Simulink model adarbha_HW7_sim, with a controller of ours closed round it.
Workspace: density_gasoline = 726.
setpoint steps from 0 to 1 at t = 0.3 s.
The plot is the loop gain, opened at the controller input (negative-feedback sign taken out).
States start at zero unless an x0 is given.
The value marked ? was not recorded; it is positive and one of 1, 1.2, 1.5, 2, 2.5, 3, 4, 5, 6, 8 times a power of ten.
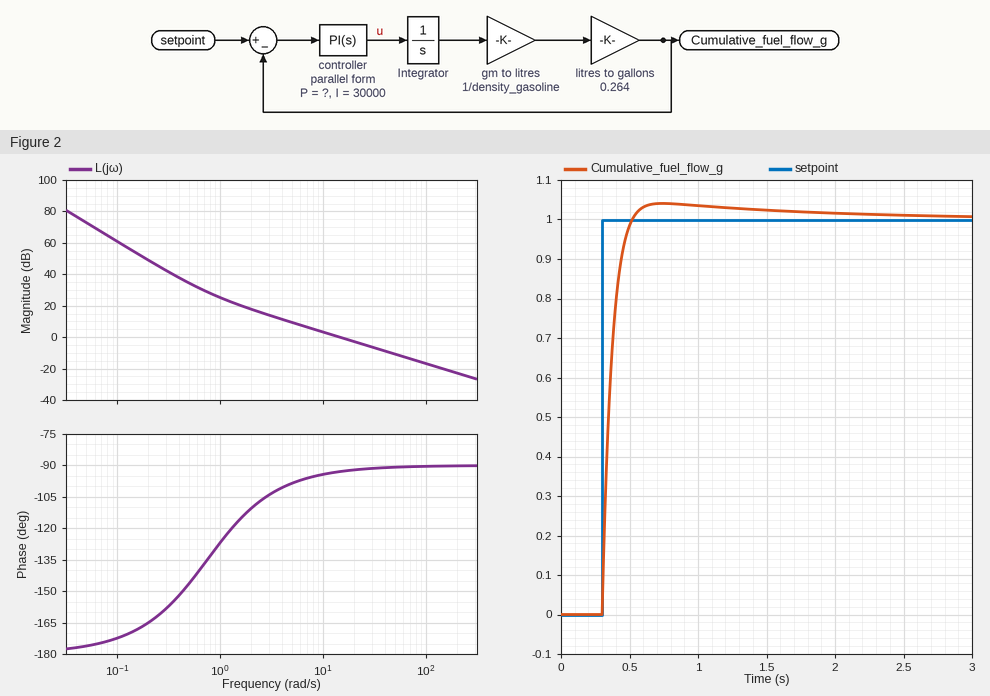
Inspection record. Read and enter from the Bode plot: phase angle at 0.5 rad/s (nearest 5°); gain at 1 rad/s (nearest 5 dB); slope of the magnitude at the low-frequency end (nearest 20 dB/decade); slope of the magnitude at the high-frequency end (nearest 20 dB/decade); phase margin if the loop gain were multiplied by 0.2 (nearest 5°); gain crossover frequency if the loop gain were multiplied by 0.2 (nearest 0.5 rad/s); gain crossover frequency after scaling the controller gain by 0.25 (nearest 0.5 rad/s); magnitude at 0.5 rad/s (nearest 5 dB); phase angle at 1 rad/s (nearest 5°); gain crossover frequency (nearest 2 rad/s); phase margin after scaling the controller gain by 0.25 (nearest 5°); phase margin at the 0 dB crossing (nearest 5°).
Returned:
-145°
25 dB
-40 dB/decade
-20 dB/decade
75°
3.0 rad/s
3.5 rad/s
35 dB
-125°
14 rad/s
80°
85°
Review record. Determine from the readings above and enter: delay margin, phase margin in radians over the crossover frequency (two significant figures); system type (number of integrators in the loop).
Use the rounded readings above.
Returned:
0.11 s
2
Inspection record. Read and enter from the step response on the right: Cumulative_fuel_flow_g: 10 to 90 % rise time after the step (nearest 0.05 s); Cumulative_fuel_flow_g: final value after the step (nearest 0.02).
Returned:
0.15 s
1.00
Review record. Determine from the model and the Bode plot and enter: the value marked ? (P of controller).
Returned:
40000
